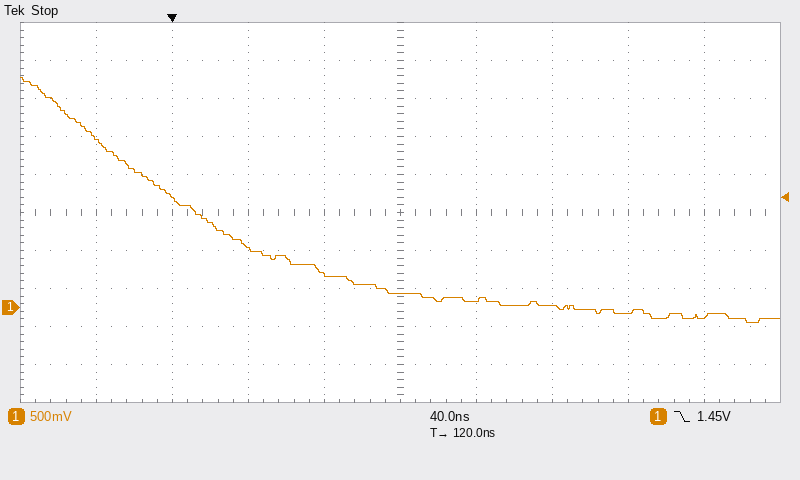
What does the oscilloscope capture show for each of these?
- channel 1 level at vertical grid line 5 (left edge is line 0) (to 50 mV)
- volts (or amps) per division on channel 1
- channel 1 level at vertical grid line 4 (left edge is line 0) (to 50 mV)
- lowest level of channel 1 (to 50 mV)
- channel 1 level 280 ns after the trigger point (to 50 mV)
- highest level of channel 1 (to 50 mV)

200 mV
500 mV
450 mV
-200 mV
-100 mV
3.05 V
